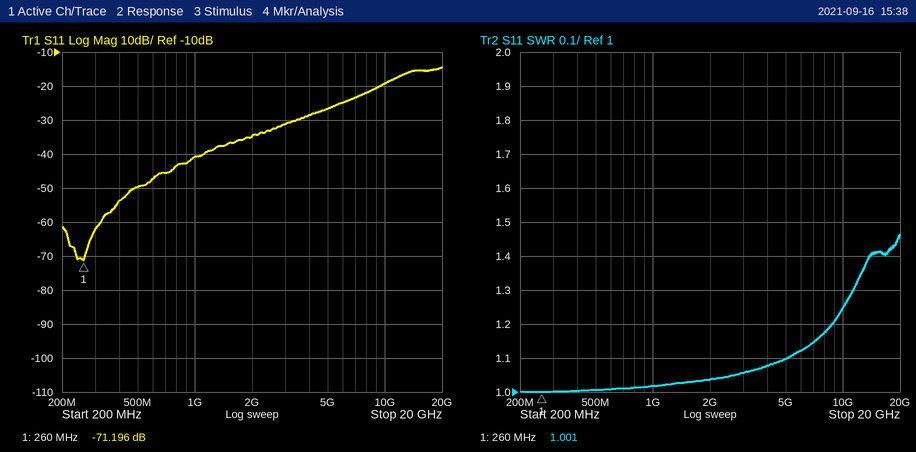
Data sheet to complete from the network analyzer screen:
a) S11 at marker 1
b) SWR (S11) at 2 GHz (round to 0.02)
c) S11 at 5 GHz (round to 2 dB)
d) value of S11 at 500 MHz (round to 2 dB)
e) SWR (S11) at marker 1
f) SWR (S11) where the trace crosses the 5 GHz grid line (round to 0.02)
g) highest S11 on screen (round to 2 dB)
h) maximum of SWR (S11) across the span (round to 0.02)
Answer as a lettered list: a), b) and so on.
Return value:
a) -71.196 dB
b) 1.04
c) -26 dB
d) -50 dB
e) 1.001
f) 1.10
g) -14 dB
h) 1.46
